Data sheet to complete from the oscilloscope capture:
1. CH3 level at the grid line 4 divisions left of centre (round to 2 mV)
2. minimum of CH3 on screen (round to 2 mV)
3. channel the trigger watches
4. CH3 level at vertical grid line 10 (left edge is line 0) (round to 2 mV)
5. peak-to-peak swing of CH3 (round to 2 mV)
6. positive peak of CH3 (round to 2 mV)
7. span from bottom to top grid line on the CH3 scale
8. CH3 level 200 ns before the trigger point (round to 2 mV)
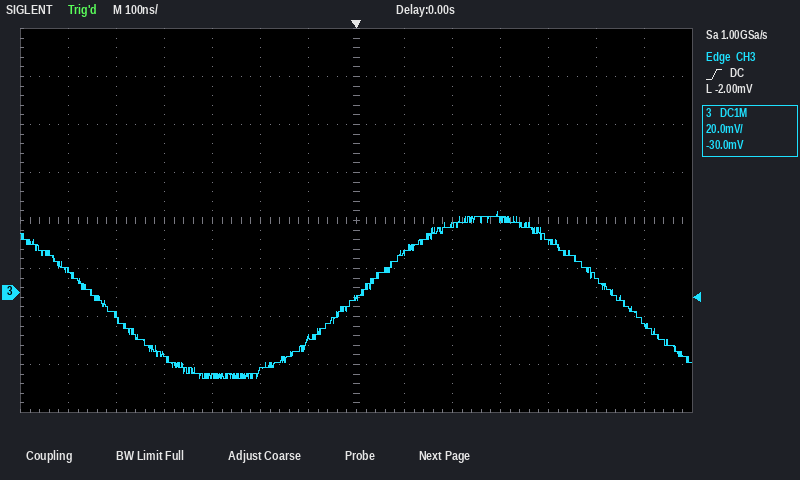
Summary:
-26 mV
-36 mV
CH3
30 mV
70 mV
34 mV
160 mV
-32 mV
